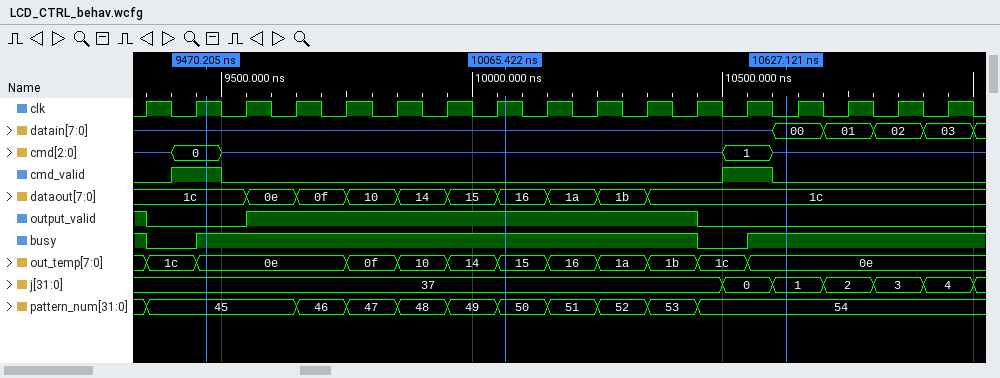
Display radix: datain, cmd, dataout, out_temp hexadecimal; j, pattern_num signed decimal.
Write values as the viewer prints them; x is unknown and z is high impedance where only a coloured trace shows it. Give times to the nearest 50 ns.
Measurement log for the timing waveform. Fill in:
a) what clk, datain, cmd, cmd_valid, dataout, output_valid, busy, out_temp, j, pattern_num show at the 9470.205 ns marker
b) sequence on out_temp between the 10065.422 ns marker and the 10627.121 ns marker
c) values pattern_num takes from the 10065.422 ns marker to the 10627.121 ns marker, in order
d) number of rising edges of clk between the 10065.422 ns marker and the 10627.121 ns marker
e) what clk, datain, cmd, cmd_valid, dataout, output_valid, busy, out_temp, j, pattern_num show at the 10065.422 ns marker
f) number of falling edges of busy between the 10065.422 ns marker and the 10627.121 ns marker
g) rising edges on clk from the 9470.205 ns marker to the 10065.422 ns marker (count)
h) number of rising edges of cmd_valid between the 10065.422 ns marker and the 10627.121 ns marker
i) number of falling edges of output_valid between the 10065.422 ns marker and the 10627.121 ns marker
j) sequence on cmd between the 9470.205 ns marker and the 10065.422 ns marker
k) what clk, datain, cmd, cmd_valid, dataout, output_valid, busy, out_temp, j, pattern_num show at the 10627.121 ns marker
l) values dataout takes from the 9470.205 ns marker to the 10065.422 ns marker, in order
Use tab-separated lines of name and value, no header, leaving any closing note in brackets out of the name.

what clk, datain, cmd, cmd_valid, dataout, output_valid, busy, out_temp, j, pattern_num show at the 9470.205 ns marker	clk=1, datain=z, cmd=0, cmd_valid=1, dataout=1c, output_valid=0, busy=1, out_temp=0e, j=37, pattern_num=45
sequence on out_temp between the 10065.422 ns marker and the 10627.121 ns marker	15, 16, 1a, 1b, 1c, 0e
values pattern_num takes from the 10065.422 ns marker to the 10627.121 ns marker, in order	50, 51, 52, 53, 54
number of rising edges of clk between the 10065.422 ns marker and the 10627.121 ns marker	5
what clk, datain, cmd, cmd_valid, dataout, output_valid, busy, out_temp, j, pattern_num show at the 10065.422 ns marker	clk=1, datain=z, cmd=z, cmd_valid=0, dataout=16, output_valid=1, busy=1, out_temp=15, j=37, pattern_num=50
number of falling edges of busy between the 10065.422 ns marker and the 10627.121 ns marker	1
rising edges on clk from the 9470.205 ns marker to the 10065.422 ns marker	6
number of rising edges of cmd_valid between the 10065.422 ns marker and the 10627.121 ns marker	1
number of falling edges of output_valid between the 10065.422 ns marker and the 10627.121 ns marker	1
sequence on cmd between the 9470.205 ns marker and the 10065.422 ns marker	0, z
what clk, datain, cmd, cmd_valid, dataout, output_valid, busy, out_temp, j, pattern_num show at the 10627.121 ns marker	clk=0, datain=00, cmd=z, cmd_valid=0, dataout=1c, output_valid=0, busy=1, out_temp=0e, j=1, pattern_num=54
values dataout takes from the 9470.205 ns marker to the 10065.422 ns marker, in order	1c, 0e, 0f, 10, 14, 15, 16
